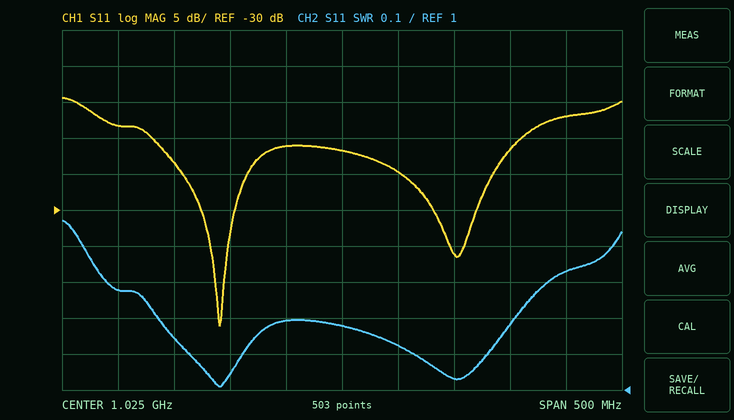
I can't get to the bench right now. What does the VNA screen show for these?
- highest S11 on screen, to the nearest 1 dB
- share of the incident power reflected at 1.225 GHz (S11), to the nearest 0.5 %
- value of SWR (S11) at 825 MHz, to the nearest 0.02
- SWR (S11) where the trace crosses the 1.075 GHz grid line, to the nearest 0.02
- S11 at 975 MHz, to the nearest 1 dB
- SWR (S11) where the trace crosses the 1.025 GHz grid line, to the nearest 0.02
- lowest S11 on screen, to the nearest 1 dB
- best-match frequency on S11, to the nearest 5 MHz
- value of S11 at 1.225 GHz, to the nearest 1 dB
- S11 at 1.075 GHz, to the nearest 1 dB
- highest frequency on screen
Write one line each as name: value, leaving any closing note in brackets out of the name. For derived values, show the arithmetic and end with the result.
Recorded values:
highest S11 on screen, to the nearest 1 dB: -14 dB
share of the incident power reflected at 1.225 GHz (S11), to the nearest 0.5 %: 10^(-17/10) ≈ 2.0 %
value of SWR (S11) at 825 MHz, to the nearest 0.02: 1.28
SWR (S11) where the trace crosses the 1.075 GHz grid line, to the nearest 0.02: 1.12
S11 at 975 MHz, to the nearest 1 dB: -21 dB
SWR (S11) where the trace crosses the 1.025 GHz grid line, to the nearest 0.02: 1.18
lowest S11 on screen, to the nearest 1 dB: -46 dB
best-match frequency on S11, to the nearest 5 MHz: 915 MHz
value of S11 at 1.225 GHz, to the nearest 1 dB: -17 dB
S11 at 1.075 GHz, to the nearest 1 dB: -25 dB
highest frequency on screen: 1.275 GHz
